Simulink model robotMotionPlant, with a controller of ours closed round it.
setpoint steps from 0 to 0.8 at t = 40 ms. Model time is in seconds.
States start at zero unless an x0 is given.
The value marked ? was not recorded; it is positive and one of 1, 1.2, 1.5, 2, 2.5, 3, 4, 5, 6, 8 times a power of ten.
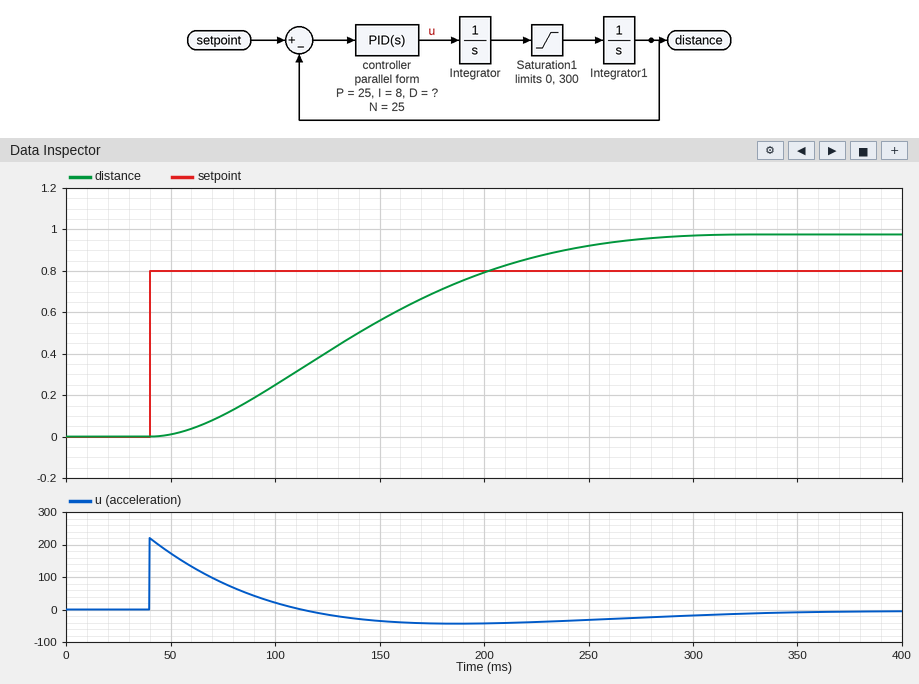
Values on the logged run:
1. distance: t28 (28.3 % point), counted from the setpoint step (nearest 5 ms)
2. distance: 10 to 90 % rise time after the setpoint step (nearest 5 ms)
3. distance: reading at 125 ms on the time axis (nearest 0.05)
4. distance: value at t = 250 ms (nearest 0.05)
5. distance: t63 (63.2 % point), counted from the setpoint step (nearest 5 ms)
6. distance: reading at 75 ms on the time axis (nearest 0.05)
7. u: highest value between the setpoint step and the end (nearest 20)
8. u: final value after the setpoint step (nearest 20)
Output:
65 ms
155 ms
0.40
0.90
120 ms
0.10
220
0
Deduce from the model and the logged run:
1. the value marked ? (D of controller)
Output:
10
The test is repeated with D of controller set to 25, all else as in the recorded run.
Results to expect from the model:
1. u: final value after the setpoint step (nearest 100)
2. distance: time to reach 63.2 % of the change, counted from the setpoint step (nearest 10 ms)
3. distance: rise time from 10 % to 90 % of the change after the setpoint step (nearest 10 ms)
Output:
0
70 ms
80 ms
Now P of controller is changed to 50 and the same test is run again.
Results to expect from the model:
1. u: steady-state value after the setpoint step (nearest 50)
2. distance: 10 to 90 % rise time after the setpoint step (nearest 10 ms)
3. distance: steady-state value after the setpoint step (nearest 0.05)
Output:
0
140 ms
1.05
